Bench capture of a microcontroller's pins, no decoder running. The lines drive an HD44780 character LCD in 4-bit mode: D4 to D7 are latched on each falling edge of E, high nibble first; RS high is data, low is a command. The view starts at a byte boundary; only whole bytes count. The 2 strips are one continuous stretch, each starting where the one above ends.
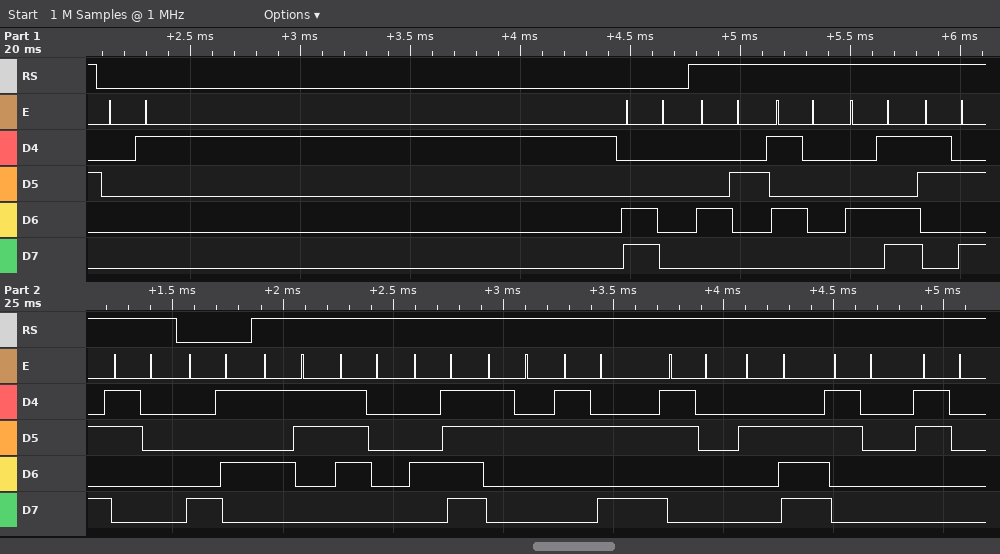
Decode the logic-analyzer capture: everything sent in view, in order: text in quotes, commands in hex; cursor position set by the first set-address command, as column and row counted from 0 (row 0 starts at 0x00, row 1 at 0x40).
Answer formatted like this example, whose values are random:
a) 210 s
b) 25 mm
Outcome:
a) 0x01 0xC0 "BPM:0" 0x85 "SpO2:0.00"
b) column 0, row 1
